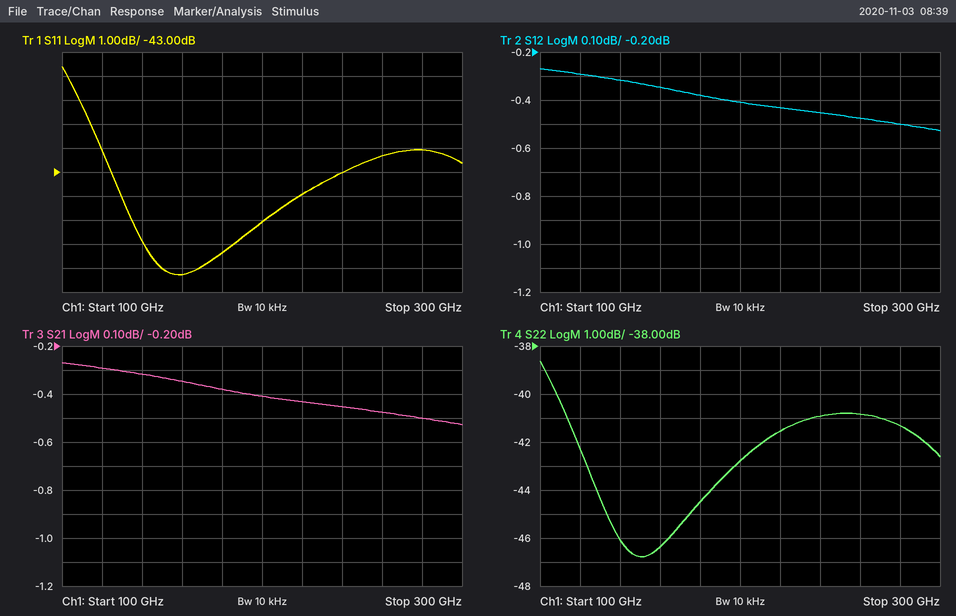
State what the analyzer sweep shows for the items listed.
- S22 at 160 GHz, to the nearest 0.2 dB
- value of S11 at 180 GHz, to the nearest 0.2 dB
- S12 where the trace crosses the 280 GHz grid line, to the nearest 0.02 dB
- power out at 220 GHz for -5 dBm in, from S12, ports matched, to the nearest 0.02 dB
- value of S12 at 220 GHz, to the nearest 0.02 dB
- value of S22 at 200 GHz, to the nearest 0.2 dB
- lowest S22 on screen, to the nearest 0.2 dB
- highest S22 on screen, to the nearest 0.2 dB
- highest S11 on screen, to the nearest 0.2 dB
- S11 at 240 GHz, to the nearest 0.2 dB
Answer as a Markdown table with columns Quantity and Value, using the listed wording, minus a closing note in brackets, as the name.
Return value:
| Quantity | Value |
|---|---|
| S22 at 160 GHz, to the nearest 0.2 dB | -46.4 dB |
| value of S11 at 180 GHz, to the nearest 0.2 dB | -46.4 dB |
| S12 where the trace crosses the 280 GHz grid line, to the nearest 0.02 dB | -0.50 dB |
| power out at 220 GHz for -5 dBm in, from S12, ports matched, to the nearest 0.02 dB | -5.44 dBm |
| value of S12 at 220 GHz, to the nearest 0.02 dB | -0.44 dB |
| value of S22 at 200 GHz, to the nearest 0.2 dB | -42.8 dB |
| lowest S22 on screen, to the nearest 0.2 dB | -46.8 dB |
| highest S22 on screen, to the nearest 0.2 dB | -38.6 dB |
| highest S11 on screen, to the nearest 0.2 dB | -38.6 dB |
| S11 at 240 GHz, to the nearest 0.2 dB | -43.0 dB |
